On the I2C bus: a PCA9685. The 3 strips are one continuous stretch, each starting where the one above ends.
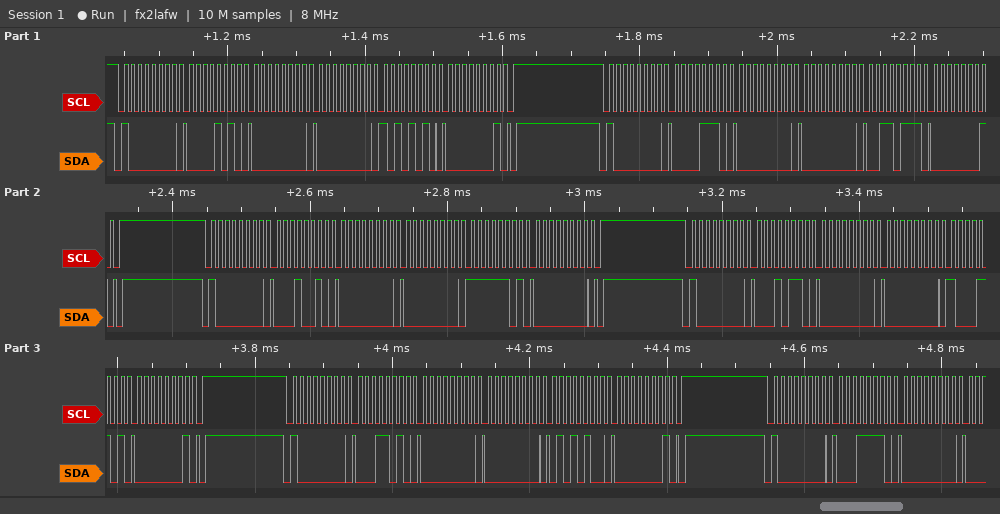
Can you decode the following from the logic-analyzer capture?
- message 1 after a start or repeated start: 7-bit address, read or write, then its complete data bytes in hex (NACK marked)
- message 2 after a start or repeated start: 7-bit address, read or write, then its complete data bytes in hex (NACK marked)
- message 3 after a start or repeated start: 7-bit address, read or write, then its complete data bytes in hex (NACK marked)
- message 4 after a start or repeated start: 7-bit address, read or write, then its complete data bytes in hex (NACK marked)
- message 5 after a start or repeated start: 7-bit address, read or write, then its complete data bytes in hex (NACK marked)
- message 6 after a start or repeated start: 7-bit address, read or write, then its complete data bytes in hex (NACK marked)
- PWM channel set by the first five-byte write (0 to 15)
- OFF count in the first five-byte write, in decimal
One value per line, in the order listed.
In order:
0x40 write: 0A 00 00 AA 01
0x40 write: 0E 00 00 37 01
0x40 write: 12 00 00 FD 00
0x40 write: 16 00 00 8D 01
0x40 write: 1A 00 00 54 01
0x40 write: 1E 00
1
426
